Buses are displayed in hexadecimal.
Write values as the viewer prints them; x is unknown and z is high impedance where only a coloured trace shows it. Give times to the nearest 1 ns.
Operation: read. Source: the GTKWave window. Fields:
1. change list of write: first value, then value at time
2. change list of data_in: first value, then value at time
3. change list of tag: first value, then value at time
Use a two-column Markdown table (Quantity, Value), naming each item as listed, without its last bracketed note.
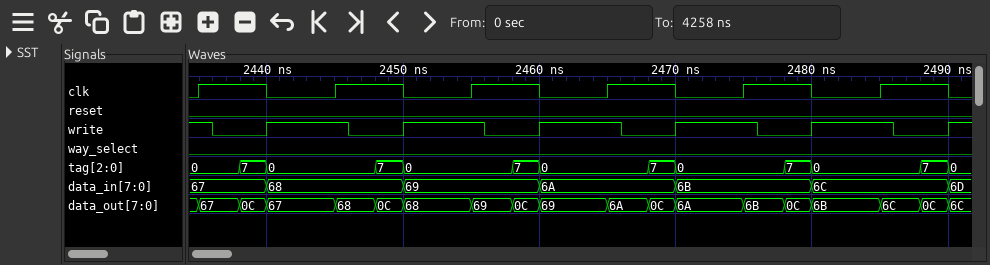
| Quantity | Value |
|---|---|
| change list of write: first value, then value at time | 1, 0 at 2436 ns, 1 at 2440 ns, 0 at 2446 ns, 1 at 2450 ns, 0 at 2456 ns, 1 at 2460 ns, 0 at 2466 ns, 1 at 2470 ns, 0 at 2476 ns, 1 at 2480 ns, 0 at 2486 ns, 1 at 2490 ns |
| change list of data_in: first value, then value at time | 67, 68 at 2440 ns, 69 at 2450 ns, 6A at 2460 ns, 6B at 2470 ns, 6C at 2480 ns, 6D at 2490 ns |
| change list of tag: first value, then value at time | 0, 7 at 2438 ns, 0 at 2440 ns, 7 at 2448 ns, 0 at 2450 ns, 7 at 2458 ns, 0 at 2460 ns, 7 at 2468 ns, 0 at 2470 ns, 7 at 2478 ns, 0 at 2480 ns, 7 at 2488 ns, 0 at 2490 ns |
